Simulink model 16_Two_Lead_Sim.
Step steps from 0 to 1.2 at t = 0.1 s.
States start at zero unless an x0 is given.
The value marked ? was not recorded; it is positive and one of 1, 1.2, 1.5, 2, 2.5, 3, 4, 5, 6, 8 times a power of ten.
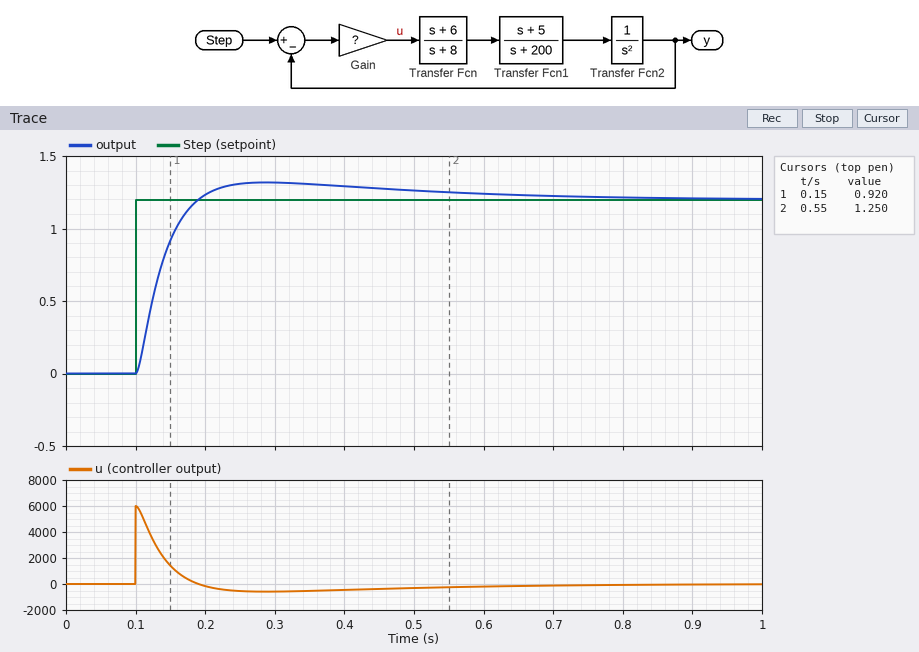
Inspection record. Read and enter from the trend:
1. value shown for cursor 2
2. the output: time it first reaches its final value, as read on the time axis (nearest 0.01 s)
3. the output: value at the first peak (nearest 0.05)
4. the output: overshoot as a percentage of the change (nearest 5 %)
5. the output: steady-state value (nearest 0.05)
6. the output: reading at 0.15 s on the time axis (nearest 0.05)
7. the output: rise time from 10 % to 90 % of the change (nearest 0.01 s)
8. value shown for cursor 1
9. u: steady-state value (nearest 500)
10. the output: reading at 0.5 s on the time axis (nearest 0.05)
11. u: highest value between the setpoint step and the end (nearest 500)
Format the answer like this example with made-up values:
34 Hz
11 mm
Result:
1.250
0.19 s
1.30
10 %
1.20
0.90
0.06 s
0.920
0
1.25
6000
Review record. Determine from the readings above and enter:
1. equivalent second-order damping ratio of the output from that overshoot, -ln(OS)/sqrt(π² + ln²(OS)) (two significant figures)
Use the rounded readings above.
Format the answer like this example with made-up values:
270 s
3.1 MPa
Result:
0.59
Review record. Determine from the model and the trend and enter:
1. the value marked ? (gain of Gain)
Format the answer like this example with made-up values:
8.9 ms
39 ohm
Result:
5000
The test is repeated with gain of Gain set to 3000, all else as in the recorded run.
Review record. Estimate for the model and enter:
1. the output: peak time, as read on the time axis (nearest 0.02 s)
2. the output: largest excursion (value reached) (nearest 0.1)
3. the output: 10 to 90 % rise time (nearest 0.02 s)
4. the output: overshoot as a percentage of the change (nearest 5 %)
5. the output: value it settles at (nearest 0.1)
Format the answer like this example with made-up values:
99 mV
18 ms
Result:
0.38 s
1.4
0.10 s
15 %
1.2
